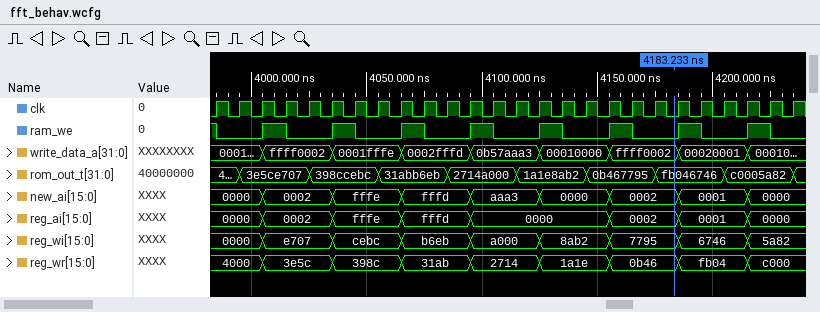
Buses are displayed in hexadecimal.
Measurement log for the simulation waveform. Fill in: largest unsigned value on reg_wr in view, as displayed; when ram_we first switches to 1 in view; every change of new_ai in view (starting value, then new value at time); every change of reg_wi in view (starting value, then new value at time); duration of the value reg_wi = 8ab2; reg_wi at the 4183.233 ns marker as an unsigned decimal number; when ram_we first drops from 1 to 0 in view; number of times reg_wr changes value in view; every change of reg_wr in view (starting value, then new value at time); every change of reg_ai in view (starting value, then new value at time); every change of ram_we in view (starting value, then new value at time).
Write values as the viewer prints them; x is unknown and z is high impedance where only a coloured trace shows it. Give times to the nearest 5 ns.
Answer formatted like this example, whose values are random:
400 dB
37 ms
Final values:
fb04
4005 ns
0000, 0002 at 4005 ns, fffe at 4035 ns, fffd at 4065 ns, aaa3 at 4095 ns, 0000 at 4125 ns, 0002 at 4155 ns, 0001 at 4185 ns, 0000 at 4215 ns
0000, e707 at 4005 ns, cebc at 4035 ns, b6eb at 4065 ns, a000 at 4095 ns, 8ab2 at 4125 ns, 7795 at 4155 ns, 6746 at 4185 ns, 5a82 at 4215 ns
30 ns
30613
3985 ns
8
4000, 3e5c at 4005 ns, 398c at 4035 ns, 31ab at 4065 ns, 2714 at 4095 ns, 1a1e at 4125 ns, 0b46 at 4155 ns, fb04 at 4185 ns, c000 at 4215 ns
0000, 0002 at 4005 ns, fffe at 4035 ns, fffd at 4065 ns, 0000 at 4095 ns, 0002 at 4155 ns, 0001 at 4185 ns, 0000 at 4215 ns
1, 0 at 3985 ns, 1 at 4005 ns, 0 at 4015 ns, 1 at 4035 ns, 0 at 4045 ns, 1 at 4065 ns, 0 at 4075 ns, 1 at 4095 ns, 0 at 4105 ns, 1 at 4125 ns, 0 at 4135 ns, 1 at 4155 ns, 0 at 4165 ns, 1 at 4185 ns, 0 at 4195 ns, 1 at 4215 ns, 0 at 4225 ns
